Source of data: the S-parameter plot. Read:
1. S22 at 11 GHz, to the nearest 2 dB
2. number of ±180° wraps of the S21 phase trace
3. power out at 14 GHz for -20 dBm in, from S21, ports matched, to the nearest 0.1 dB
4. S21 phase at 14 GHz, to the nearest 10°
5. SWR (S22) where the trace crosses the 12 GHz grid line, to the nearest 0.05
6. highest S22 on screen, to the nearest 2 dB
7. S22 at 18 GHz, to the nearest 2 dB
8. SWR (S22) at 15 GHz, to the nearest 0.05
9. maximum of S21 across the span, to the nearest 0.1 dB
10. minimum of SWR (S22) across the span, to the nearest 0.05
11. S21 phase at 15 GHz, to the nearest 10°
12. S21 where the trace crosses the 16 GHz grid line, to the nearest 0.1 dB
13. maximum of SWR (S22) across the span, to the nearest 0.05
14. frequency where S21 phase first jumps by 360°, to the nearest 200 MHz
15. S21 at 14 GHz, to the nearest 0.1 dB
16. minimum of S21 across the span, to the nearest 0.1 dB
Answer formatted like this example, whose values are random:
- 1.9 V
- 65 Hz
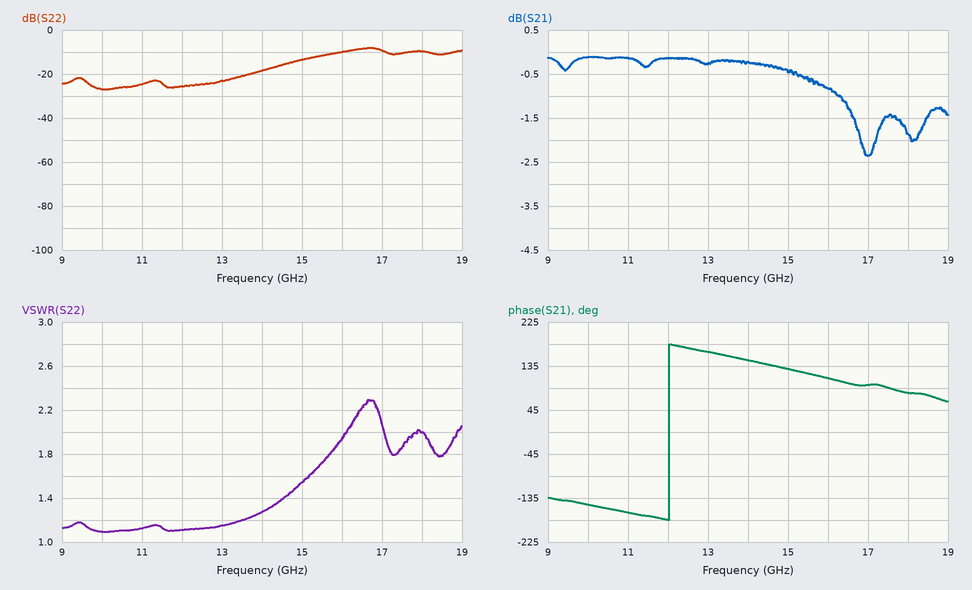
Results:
- -24 dB
- 1
- -20.2 dBm
- 150°
- 1.10
- -8 dB
- -10 dB
- 1.55
- -0.1 dB
- 1.10
- 130°
- -0.8 dB
- 2.30
- 12.0 GHz
- -0.2 dB
- -2.4 dB
